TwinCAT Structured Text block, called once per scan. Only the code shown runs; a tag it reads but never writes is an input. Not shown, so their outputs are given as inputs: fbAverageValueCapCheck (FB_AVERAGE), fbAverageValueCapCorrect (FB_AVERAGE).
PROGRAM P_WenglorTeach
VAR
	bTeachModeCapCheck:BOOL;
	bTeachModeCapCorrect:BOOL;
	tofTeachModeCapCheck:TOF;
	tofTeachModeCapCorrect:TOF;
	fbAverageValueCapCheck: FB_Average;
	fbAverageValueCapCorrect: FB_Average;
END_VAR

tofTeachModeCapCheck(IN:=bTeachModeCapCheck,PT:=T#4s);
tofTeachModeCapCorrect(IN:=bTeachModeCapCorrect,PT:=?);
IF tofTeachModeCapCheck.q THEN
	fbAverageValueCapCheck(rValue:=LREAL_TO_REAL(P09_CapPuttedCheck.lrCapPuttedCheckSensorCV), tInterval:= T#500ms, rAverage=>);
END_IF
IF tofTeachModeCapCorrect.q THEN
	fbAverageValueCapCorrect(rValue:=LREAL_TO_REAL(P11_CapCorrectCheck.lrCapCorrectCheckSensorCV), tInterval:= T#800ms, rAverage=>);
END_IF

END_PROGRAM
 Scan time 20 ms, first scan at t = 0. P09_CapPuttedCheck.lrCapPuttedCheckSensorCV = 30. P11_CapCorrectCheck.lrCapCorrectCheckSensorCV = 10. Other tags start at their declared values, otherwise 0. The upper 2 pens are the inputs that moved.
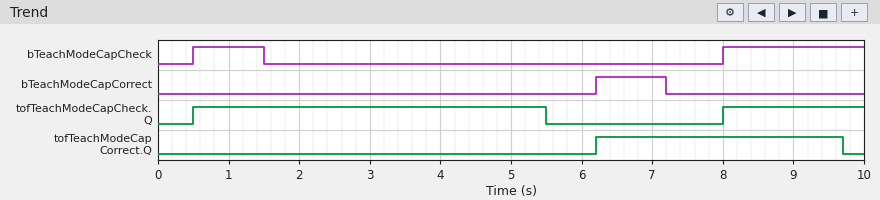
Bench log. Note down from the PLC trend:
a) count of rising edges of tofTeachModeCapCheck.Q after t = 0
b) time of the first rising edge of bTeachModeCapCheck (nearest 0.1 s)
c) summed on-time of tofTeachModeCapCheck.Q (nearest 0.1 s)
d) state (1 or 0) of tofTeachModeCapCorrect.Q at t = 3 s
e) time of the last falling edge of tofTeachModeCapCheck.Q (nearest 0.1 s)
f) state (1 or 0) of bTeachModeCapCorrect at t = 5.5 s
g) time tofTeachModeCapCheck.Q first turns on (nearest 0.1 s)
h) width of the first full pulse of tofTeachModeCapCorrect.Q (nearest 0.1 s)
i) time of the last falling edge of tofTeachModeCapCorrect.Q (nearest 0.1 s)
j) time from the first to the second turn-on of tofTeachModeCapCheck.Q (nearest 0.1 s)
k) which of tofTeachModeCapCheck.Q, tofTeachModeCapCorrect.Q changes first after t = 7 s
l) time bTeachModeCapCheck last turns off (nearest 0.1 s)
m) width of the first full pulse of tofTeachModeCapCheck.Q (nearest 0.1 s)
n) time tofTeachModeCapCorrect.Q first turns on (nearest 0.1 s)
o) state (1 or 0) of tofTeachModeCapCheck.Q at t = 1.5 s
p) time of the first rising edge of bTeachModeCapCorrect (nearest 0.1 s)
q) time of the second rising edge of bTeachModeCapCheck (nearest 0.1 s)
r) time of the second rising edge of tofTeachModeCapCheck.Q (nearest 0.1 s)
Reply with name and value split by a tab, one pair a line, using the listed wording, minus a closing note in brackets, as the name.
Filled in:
count of rising edges of tofTeachModeCapCheck.Q after t = 0	2
time of the first rising edge of bTeachModeCapCheck	0.5 s
summed on-time of tofTeachModeCapCheck.Q	7.0 s
state (1 or 0) of tofTeachModeCapCorrect.Q at t = 3 s	0
time of the last falling edge of tofTeachModeCapCheck.Q	5.5 s
state (1 or 0) of bTeachModeCapCorrect at t = 5.5 s	0
time tofTeachModeCapCheck.Q first turns on	0.5 s
width of the first full pulse of tofTeachModeCapCorrect.Q	3.5 s
time of the last falling edge of tofTeachModeCapCorrect.Q	9.7 s
time from the first to the second turn-on of tofTeachModeCapCheck.Q	7.5 s
which of tofTeachModeCapCheck.Q, tofTeachModeCapCorrect.Q changes first after t = 7 s	tofTeachModeCapCheck.Q
time bTeachModeCapCheck last turns off	1.5 s
width of the first full pulse of tofTeachModeCapCheck.Q	5.0 s
time tofTeachModeCapCorrect.Q first turns on	6.2 s
state (1 or 0) of tofTeachModeCapCheck.Q at t = 1.5 s	1
time of the first rising edge of bTeachModeCapCorrect	6.2 s
time of the second rising edge of bTeachModeCapCheck	8.0 s
time of the second rising edge of tofTeachModeCapCheck.Q	8.0 s
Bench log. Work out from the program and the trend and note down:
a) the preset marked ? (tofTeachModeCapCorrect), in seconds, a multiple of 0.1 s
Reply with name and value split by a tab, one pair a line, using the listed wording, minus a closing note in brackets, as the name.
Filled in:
the preset marked ? (tofTeachModeCapCorrect), in seconds, a multiple of 0.1 s	2.5 s
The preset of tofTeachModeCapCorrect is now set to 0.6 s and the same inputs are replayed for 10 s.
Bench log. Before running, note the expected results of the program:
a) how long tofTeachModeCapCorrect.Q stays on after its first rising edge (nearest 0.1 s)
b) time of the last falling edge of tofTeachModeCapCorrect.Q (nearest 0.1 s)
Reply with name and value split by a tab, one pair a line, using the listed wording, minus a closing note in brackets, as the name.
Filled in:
how long tofTeachModeCapCorrect.Q stays on after its first rising edge	1.6 s
time of the last falling edge of tofTeachModeCapCorrect.Q	7.8 s
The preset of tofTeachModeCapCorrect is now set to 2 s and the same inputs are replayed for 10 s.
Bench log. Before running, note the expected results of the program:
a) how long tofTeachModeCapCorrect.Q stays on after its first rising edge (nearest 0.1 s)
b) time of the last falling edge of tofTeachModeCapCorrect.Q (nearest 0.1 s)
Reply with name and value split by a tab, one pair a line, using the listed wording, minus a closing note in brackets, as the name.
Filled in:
how long tofTeachModeCapCorrect.Q stays on after its first rising edge	3.0 s
time of the last falling edge of tofTeachModeCapCorrect.Q	9.2 s
